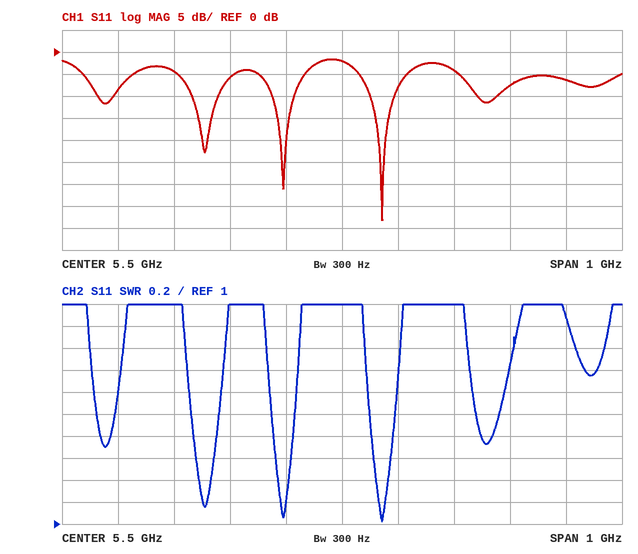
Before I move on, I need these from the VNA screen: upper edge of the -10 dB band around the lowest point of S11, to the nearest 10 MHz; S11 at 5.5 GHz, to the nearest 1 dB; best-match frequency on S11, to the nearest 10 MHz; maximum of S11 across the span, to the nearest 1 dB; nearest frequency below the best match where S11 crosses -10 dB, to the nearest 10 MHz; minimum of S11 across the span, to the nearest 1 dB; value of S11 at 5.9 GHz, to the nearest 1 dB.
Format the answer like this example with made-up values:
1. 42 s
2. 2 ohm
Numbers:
1. 5.59 GHz
2. -2 dB
3. 5.57 GHz
4. -2 dB
5. 5.55 GHz
6. -38 dB
7. -6 dB
